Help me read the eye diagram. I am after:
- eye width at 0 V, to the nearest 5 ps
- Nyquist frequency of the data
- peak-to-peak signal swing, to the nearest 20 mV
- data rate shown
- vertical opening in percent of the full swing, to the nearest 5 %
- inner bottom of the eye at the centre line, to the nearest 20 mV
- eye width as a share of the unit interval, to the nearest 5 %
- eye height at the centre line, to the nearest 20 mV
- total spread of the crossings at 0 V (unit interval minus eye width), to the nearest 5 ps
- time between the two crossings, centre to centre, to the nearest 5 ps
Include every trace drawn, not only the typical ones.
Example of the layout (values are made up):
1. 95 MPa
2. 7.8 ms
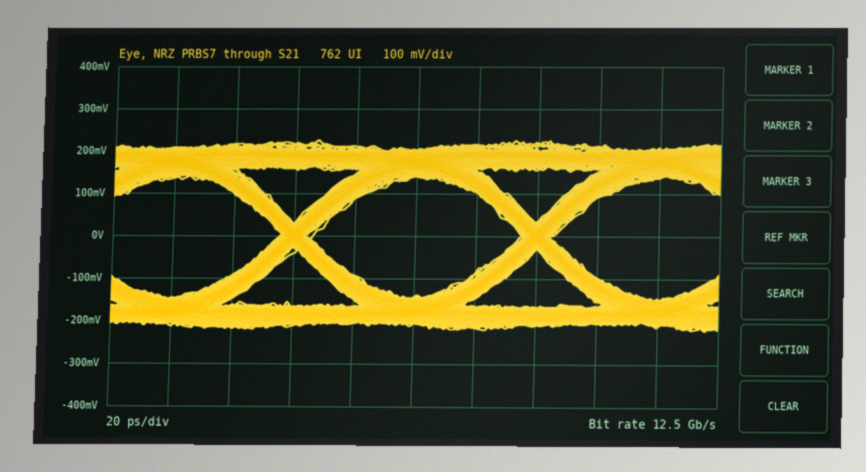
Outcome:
1. 70 ps
2. 6.25 GHz
3. 440 mV
4. 12.5 Gb/s
5. 65 %
6. -140 mV
7. 85 %
8. 280 mV
9. 10 ps
10. 80 ps
